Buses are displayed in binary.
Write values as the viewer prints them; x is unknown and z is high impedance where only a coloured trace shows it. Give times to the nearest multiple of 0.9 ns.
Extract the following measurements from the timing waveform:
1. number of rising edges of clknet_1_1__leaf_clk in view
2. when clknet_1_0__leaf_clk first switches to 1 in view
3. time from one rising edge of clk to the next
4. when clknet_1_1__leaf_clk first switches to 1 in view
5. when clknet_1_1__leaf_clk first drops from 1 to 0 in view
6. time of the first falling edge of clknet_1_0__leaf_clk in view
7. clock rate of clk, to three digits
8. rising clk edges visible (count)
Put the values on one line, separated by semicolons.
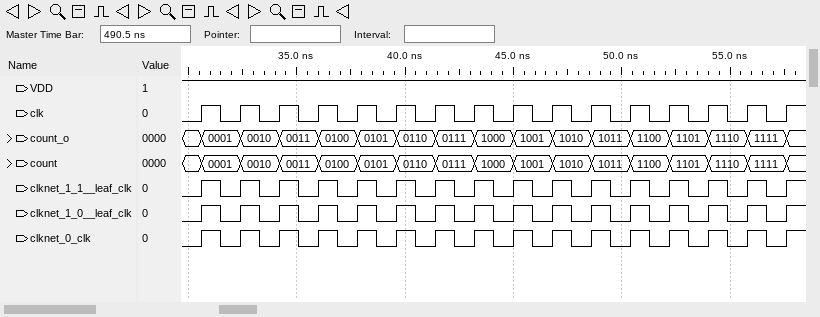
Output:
16; 30.6 ns; 1.8 ns; 30.6 ns; 31.5 ns; 31.5 ns; 556 MHz; 16
